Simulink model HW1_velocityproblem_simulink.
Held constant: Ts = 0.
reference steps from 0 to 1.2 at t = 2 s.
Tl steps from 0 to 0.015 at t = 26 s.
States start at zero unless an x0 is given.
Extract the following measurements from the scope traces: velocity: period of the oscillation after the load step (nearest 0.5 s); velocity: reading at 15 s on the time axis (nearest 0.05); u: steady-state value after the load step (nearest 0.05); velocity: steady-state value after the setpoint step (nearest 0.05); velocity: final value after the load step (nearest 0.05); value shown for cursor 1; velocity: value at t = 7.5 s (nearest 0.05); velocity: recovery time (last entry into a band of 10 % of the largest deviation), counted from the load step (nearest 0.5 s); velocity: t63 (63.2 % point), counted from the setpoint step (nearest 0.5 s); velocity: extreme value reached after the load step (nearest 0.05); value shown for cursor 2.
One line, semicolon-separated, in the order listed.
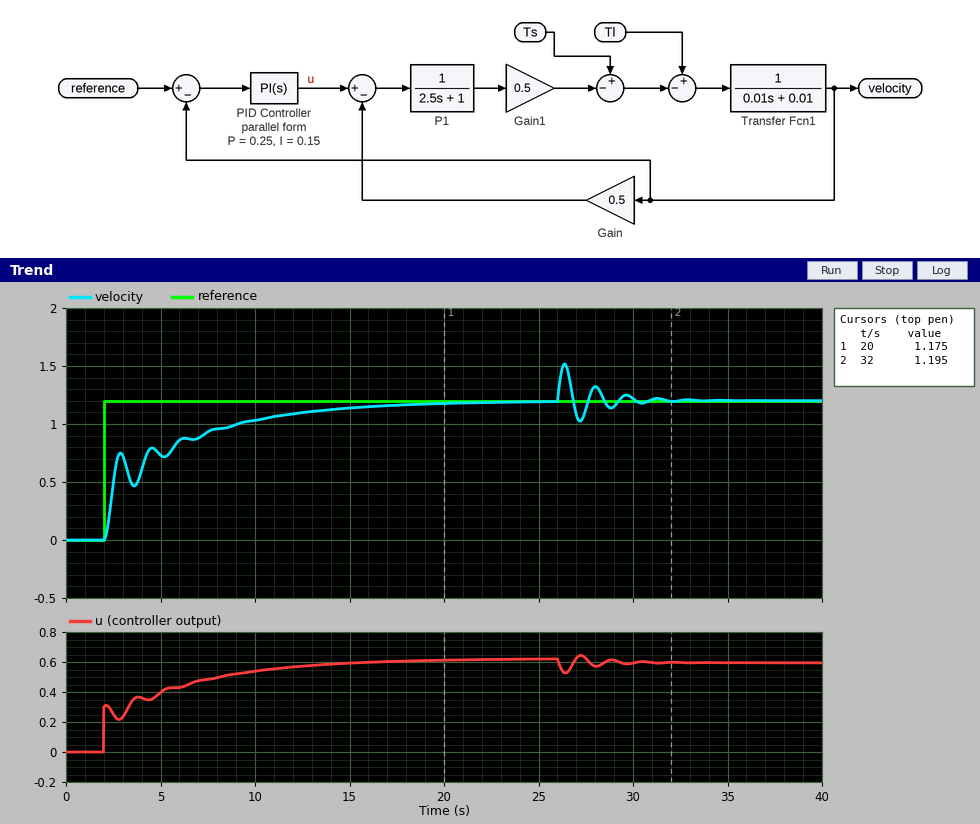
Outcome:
1.5 s; 1.15; 0.60; 1.20; 1.20; 1.175; 0.95; 4.0 s; 2.5 s; 1.50; 1.195
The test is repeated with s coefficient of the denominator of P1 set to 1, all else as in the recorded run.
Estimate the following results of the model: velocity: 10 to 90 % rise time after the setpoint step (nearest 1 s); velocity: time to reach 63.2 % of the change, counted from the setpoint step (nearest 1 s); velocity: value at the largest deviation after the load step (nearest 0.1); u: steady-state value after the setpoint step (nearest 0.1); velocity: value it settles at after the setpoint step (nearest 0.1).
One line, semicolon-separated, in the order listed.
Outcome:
10 s; 3 s; 1.4; 0.6; 1.2
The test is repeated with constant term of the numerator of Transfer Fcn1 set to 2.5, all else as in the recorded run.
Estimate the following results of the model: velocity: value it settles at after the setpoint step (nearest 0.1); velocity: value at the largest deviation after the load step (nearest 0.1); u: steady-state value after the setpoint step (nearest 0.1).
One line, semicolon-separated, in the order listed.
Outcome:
1.2; 1.7; 0.6
